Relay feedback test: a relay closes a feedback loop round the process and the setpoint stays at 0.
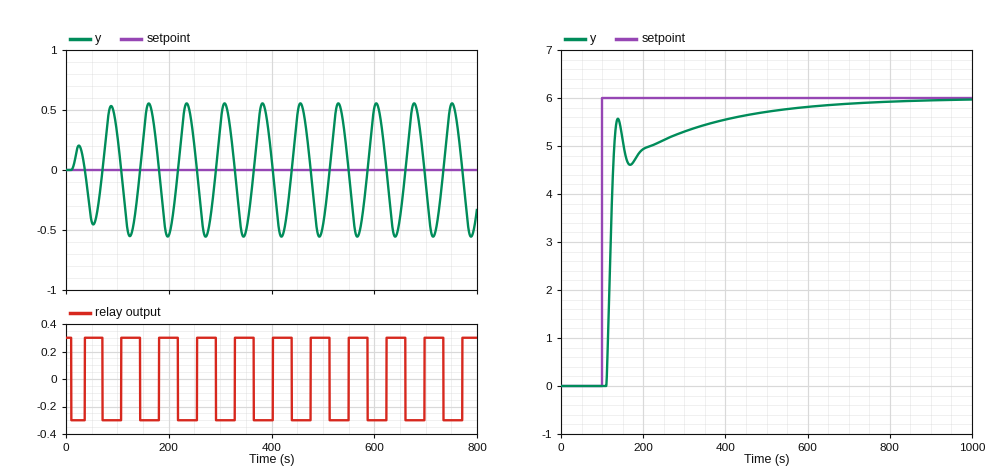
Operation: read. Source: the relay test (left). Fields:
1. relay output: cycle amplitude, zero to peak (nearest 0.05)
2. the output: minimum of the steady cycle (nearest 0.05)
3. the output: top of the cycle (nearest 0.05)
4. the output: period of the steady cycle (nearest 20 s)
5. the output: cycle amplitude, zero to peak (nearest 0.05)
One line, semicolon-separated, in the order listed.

0.30; -0.55; 0.55; 80 s; 0.55
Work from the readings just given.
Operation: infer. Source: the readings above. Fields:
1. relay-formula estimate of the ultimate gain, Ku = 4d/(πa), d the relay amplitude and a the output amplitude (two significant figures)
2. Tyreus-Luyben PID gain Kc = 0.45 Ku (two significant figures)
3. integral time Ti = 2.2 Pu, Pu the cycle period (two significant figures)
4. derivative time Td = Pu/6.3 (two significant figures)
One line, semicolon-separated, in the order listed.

0.69; 0.31; 180 s; 13 s
